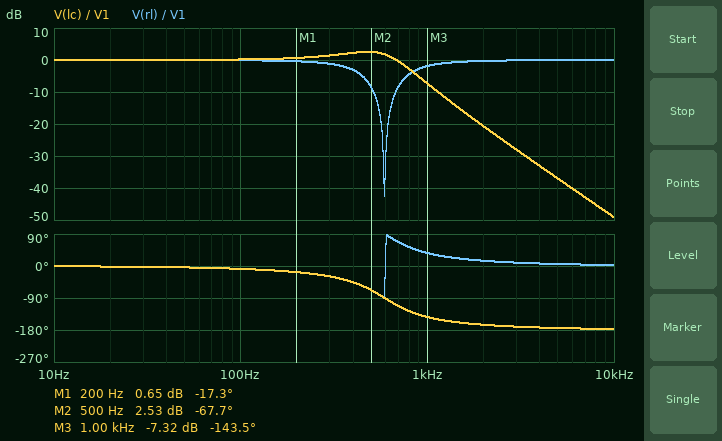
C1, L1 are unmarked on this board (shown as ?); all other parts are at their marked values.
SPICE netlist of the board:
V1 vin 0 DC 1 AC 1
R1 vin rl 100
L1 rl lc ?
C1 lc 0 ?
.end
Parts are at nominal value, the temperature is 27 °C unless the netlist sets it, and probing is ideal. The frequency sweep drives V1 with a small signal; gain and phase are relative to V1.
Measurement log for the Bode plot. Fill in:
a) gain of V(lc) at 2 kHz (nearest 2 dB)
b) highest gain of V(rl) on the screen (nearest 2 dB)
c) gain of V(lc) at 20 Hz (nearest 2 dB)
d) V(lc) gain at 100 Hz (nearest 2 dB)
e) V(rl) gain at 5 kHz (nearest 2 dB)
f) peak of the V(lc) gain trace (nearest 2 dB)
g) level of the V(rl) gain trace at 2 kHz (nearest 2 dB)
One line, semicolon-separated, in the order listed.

-20 dB; 0 dB; 0 dB; 0 dB; 0 dB; 2 dB; 0 dB
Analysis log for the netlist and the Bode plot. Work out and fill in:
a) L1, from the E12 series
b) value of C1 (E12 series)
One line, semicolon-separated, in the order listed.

33 mH; 2.2 µF
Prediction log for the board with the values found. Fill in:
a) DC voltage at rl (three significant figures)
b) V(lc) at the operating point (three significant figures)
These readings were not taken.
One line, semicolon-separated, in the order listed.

1.00 V; 1.00 V
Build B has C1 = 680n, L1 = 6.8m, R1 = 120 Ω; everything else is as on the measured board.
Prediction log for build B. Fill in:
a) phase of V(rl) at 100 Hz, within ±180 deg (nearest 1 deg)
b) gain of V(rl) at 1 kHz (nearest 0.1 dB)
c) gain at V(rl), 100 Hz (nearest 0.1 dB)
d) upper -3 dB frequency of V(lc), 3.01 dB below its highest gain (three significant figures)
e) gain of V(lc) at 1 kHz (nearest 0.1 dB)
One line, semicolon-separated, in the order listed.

-3 deg; -1.4 dB; 0 dB; 2.61 kHz; 0.3 dB
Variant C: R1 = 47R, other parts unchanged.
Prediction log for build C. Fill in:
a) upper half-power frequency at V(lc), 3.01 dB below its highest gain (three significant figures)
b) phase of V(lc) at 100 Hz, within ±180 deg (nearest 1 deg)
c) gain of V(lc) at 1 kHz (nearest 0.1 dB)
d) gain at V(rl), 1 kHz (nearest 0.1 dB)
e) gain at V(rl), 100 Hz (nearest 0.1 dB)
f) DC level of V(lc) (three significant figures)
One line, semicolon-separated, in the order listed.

674 Hz; -4 deg; -5.9 dB; -0.5 dB; 0 dB; 1.00 V
